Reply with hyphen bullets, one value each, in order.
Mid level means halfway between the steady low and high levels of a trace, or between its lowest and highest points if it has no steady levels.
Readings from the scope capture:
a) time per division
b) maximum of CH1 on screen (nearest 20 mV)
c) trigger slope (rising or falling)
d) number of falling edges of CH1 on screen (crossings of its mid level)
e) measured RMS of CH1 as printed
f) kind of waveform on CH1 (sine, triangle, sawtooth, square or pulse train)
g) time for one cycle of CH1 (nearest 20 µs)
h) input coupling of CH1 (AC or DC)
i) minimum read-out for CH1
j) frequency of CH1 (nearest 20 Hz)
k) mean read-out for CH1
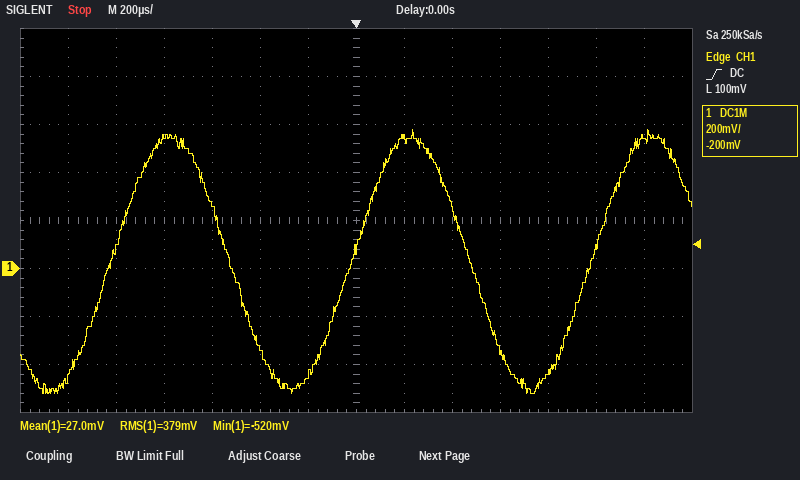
- 200 µs
- 580 mV
- rising
- 2
- 379 mV
- sine
- 1.00 ms
- DC
- -520 mV
- 1.00 kHz
- 27.0 mV
